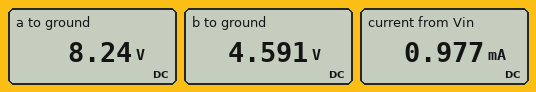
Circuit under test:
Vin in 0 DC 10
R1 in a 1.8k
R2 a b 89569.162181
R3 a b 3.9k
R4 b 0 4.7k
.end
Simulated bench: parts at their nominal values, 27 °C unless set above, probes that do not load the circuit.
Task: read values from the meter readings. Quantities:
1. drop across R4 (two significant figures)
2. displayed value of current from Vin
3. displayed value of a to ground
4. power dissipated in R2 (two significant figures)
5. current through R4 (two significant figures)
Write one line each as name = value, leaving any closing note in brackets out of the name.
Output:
drop across R4 = 4.6 V
displayed value of current from Vin = 0.977 mA
displayed value of a to ground = 8.24 V
power dissipated in R2 = 150 µW
current through R4 = 980 µA
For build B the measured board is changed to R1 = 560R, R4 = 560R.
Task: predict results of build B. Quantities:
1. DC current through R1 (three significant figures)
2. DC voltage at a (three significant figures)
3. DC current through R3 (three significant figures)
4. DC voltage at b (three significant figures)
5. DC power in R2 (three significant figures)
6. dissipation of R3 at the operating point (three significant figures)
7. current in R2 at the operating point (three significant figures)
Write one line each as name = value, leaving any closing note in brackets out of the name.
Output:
DC current through R1 = 2.06 mA
DC voltage at a = 8.85 V
DC current through R3 = 1.97 mA
DC voltage at b = 1.15 V
DC power in R2 = 661 µW
dissipation of R3 at the operating point = 15.2 mW
current in R2 at the operating point = 85.9 µA
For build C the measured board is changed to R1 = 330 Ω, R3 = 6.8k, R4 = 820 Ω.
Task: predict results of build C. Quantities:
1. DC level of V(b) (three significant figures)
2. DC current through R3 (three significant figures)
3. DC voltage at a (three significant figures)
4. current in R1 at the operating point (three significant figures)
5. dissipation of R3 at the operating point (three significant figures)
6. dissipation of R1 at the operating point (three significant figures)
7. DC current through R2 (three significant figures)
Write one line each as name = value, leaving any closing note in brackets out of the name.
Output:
DC level of V(b) = 1.10 V
DC current through R3 = 1.24 mA
DC voltage at a = 9.56 V
current in R1 at the operating point = 1.34 mA
dissipation of R3 at the operating point = 10.5 mW
dissipation of R1 at the operating point = 591 µW
DC current through R2 = 94.5 µA
